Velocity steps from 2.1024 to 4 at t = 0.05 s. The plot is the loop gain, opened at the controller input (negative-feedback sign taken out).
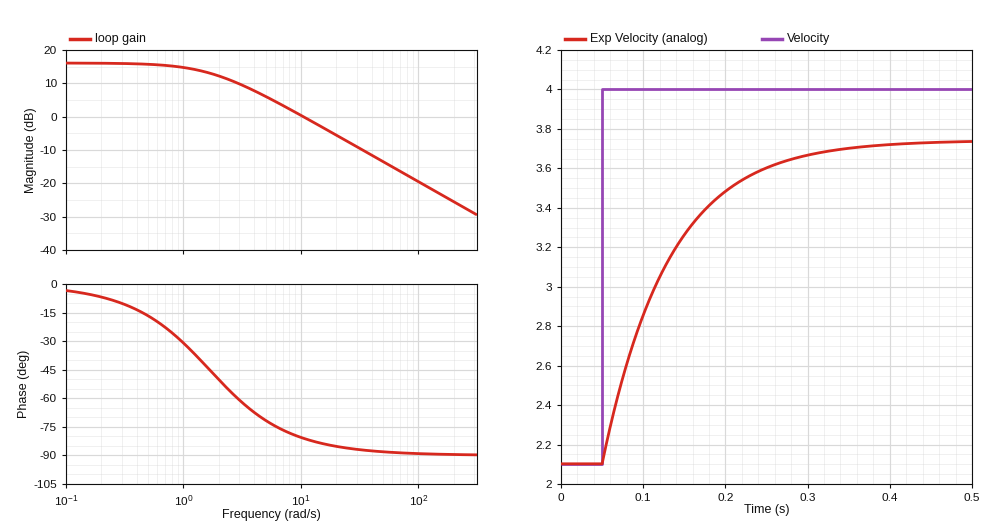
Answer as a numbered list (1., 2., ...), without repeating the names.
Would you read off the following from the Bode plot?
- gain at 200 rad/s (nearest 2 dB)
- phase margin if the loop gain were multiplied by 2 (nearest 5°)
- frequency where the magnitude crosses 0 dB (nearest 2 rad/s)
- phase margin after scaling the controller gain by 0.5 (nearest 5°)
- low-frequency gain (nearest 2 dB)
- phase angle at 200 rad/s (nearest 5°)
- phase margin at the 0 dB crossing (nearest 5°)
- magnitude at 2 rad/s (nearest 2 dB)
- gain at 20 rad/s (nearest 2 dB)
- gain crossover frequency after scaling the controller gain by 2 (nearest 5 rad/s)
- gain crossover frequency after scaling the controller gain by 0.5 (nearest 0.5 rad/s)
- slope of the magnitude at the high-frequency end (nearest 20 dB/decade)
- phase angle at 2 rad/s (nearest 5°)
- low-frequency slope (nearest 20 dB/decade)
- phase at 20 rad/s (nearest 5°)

1. -26 dB
2. 95°
3. 10 rad/s
4. 110°
5. 16 dB
6. -90°
7. 100°
8. 12 dB
9. -6 dB
10. 20 rad/s
11. 5.0 rad/s
12. -20 dB/decade
13. -50°
14. 0 dB/decade
15. -85°
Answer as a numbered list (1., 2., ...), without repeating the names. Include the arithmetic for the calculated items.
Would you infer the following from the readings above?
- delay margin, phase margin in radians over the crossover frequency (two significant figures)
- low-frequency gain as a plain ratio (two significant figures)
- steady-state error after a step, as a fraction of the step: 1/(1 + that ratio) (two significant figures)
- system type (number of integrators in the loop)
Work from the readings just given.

1. 100 × π / 180 / 10 = 0.17 s
2. 10^(16 / 20) = 6.3
3. 1 / (1 + 6.3) = 0.14
4. 0
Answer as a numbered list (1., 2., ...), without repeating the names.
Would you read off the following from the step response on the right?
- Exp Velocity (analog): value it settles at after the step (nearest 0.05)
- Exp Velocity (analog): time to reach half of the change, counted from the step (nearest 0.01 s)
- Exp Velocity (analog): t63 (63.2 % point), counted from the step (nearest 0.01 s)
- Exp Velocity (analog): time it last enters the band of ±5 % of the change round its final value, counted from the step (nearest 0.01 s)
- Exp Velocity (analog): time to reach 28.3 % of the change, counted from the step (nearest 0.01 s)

1. 3.75
2. 0.06 s
3. 0.08 s
4. 0.24 s
5. 0.03 s
